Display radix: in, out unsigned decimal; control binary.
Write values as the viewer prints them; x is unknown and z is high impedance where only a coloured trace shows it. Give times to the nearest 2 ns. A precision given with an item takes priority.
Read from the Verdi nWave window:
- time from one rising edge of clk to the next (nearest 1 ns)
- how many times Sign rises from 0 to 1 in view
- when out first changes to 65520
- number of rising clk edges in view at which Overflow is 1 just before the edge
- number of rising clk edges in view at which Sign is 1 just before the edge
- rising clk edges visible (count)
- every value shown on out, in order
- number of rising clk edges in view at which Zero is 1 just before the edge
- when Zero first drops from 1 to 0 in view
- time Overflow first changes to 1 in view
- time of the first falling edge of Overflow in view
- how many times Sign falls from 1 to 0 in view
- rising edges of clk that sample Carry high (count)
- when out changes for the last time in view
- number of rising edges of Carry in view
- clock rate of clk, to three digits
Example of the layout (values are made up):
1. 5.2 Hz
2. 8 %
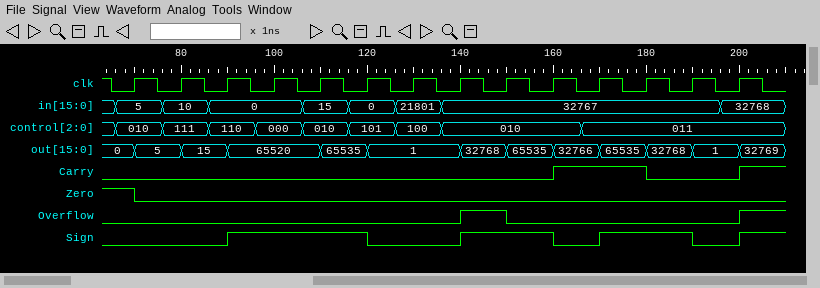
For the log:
1. 10 ns
2. 4
3. 90 ns
4. 1
5. 7
6. 14
7. 0, 5, 15, 65520, 65535, 1, 32768, 65535, 32766, 65535, 32768, 1, 32769
8. 1
9. 70 ns
10. 140 ns
11. 150 ns
12. 3
13. 2
14. 200 ns
15. 2
16. 100 MHz
